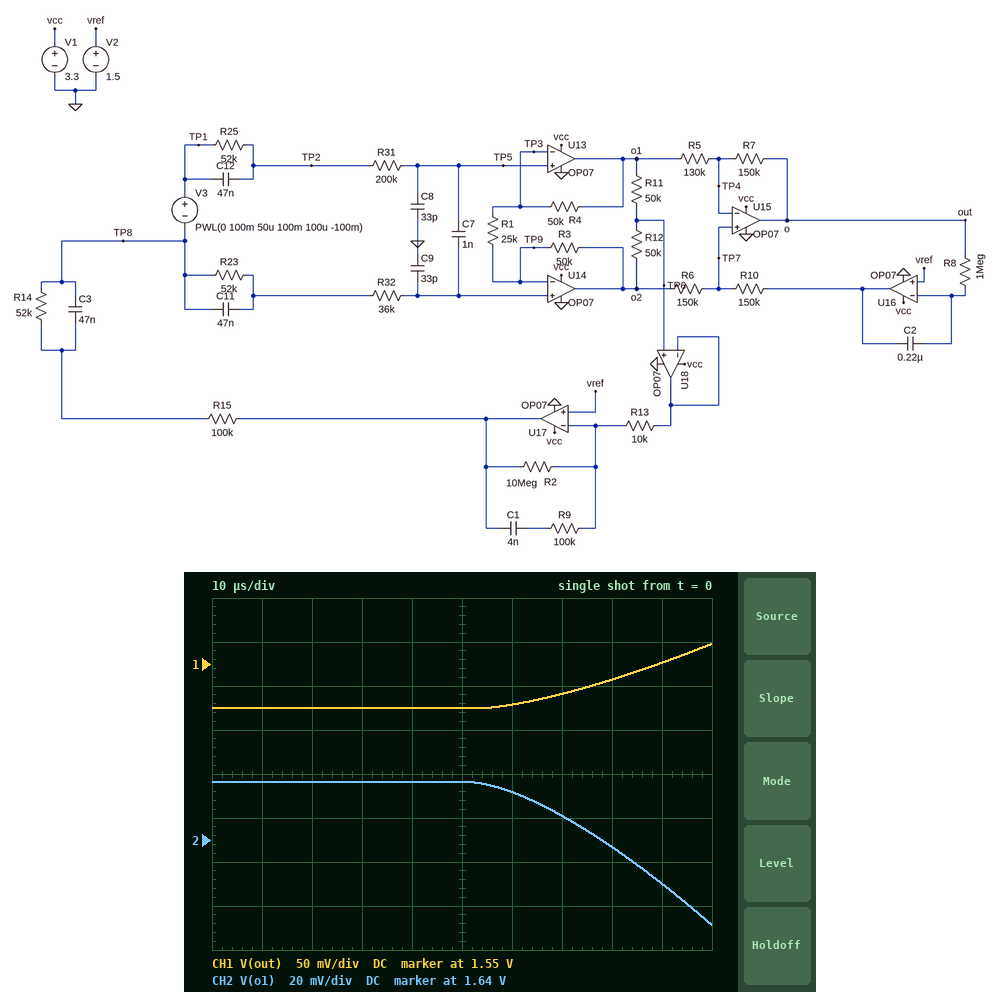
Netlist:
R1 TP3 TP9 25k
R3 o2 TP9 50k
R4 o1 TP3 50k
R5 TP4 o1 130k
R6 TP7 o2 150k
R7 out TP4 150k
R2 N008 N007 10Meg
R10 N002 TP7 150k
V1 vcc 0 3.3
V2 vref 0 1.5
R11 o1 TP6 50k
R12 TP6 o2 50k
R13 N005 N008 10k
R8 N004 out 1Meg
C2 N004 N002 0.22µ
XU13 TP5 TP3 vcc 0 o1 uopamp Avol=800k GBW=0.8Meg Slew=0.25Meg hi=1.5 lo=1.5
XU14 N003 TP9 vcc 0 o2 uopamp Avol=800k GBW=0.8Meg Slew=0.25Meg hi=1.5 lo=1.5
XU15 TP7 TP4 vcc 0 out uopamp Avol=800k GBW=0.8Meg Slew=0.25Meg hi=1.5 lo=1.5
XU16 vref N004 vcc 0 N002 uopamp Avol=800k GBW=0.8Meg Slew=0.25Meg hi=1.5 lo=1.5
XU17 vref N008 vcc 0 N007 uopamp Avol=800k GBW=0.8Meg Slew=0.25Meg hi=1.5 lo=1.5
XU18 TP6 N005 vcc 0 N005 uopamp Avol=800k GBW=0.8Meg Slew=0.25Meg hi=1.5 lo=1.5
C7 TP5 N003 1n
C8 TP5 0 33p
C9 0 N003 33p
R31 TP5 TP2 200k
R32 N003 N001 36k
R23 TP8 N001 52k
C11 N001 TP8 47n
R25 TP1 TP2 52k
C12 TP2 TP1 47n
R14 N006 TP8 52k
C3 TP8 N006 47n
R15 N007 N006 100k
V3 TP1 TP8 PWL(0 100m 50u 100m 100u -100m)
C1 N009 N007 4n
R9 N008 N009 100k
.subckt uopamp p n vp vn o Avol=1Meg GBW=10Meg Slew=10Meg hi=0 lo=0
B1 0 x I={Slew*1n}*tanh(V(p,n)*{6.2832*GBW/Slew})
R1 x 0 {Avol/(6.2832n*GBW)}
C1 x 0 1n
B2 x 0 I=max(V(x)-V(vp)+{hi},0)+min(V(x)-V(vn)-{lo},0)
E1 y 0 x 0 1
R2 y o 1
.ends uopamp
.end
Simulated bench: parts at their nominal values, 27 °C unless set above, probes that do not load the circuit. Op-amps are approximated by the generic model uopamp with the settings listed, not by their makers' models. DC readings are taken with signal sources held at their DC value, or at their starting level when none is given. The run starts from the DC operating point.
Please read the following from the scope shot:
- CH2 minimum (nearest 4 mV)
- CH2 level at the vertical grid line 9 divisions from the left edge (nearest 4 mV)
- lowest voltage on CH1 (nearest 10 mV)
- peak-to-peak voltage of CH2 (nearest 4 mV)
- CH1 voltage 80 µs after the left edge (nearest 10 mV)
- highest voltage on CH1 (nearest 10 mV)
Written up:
1.600 V
1.620 V
1.50 V
64 mV
1.53 V
1.57 V
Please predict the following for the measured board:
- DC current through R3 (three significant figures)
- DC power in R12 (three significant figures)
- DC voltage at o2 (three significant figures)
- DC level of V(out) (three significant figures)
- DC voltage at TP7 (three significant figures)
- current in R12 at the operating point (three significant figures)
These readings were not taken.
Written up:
1.33 µA
139 nW
1.50 V
1.50 V
1.59 V
1.67 µA
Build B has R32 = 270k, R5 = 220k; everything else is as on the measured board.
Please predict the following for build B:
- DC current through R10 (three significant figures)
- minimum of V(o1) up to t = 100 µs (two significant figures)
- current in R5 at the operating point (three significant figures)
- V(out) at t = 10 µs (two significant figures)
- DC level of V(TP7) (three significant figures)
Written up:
448 nA
1.5 V
450 nA
1.5 V
1.57 V
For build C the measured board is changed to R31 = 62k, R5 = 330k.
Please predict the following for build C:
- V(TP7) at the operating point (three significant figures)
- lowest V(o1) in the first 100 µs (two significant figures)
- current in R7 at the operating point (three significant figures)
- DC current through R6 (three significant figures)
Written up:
1.55 V
1.5 V
347 nA
345 nA
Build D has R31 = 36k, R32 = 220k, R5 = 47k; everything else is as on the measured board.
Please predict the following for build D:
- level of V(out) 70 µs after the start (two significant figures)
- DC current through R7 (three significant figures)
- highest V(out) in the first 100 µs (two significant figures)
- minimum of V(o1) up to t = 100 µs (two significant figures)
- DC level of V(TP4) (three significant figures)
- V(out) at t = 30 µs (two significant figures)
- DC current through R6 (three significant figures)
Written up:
1.7 V
845 nA
1.8 V
1.5 V
1.63 V
1.5 V
842 nA
